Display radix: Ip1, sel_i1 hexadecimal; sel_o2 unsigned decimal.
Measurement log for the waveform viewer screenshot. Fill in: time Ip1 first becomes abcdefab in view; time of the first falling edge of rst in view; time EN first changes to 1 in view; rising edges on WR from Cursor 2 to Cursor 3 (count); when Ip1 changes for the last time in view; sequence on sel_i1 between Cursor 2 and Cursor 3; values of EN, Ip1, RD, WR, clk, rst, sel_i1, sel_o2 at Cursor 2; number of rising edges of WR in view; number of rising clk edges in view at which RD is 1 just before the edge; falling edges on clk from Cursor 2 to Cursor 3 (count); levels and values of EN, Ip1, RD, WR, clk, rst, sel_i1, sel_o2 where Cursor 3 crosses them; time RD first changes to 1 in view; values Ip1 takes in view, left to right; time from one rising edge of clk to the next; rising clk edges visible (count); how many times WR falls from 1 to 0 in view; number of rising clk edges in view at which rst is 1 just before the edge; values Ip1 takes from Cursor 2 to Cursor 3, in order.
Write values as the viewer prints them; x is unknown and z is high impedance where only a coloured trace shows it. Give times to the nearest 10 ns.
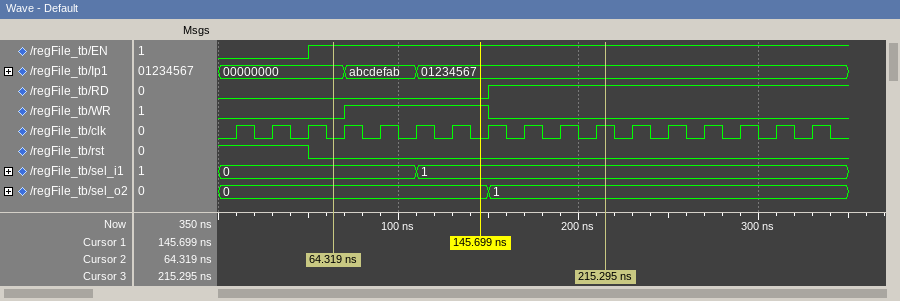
70 ns
50 ns
50 ns
1
110 ns
0, 1
EN=1, Ip1=00000000, RD=0, WR=0, clk=0, rst=0, sel_i1=0, sel_o2=0
1
9
7
EN=1, Ip1=01234567, RD=1, WR=0, clk=1, rst=0, sel_i1=1, sel_o2=1
150 ns
00000000, abcdefab, 01234567
20 ns
17
1
3
00000000, abcdefab, 01234567
